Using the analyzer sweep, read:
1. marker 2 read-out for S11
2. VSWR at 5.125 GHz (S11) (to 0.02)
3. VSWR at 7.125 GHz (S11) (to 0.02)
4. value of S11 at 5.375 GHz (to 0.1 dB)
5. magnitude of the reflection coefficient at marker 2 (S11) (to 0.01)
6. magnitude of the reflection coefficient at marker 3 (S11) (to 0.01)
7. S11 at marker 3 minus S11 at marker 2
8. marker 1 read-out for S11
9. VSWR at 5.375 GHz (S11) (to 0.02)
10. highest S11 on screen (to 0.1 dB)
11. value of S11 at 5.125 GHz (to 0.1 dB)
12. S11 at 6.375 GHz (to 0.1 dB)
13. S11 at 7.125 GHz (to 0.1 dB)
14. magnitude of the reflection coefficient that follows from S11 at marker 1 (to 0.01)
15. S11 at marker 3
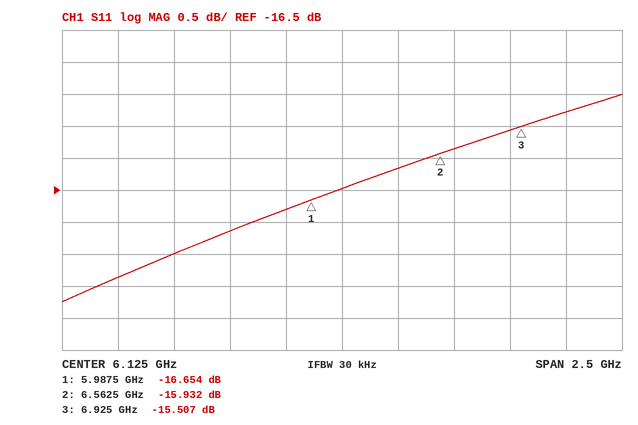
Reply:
-15.932 dB
1.30
1.42
-17.5 dB
0.16
0.17
0.425 dB
-16.654 dB
1.30
-15.0 dB
-17.9 dB
-16.2 dB
-15.3 dB
0.15
-15.507 dB
